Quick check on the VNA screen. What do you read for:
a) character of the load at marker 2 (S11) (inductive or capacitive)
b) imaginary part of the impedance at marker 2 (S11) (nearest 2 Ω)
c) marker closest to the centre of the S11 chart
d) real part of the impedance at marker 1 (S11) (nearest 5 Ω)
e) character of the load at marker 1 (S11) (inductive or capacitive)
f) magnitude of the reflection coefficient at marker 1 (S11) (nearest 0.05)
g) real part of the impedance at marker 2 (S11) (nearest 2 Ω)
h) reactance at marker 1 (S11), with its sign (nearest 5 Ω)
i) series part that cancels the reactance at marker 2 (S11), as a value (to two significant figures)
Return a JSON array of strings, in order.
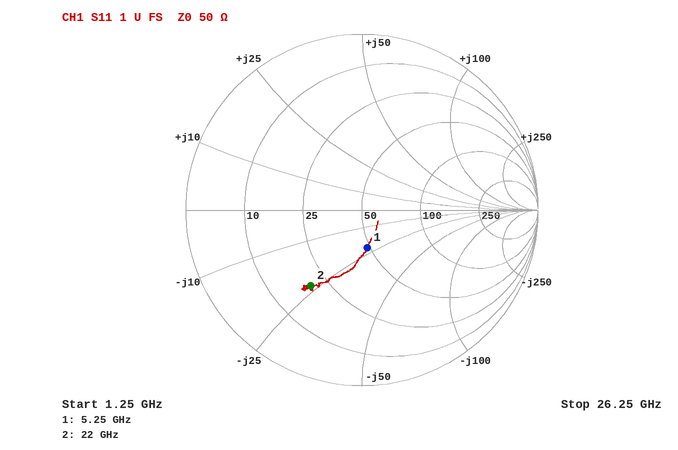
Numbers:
["capacitive", "-24 Ω", "marker 1", "50 Ω", "capacitive", "0.20", "20 Ω", "-20 Ω", "170 pH"]
